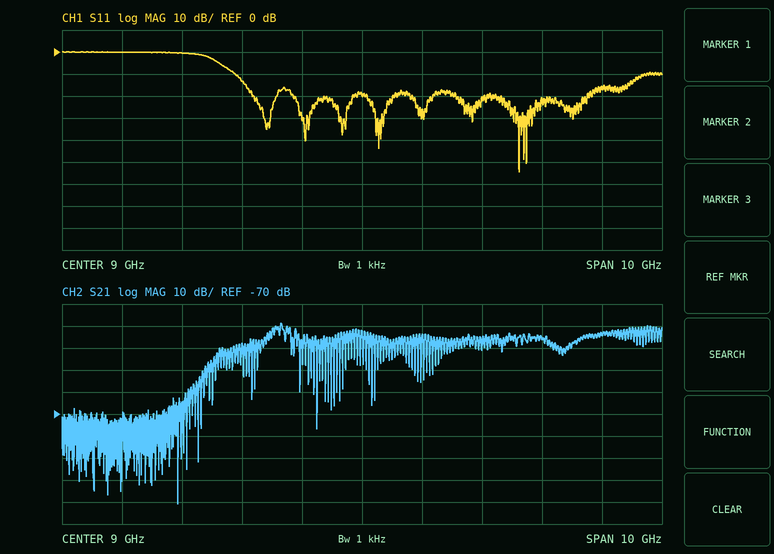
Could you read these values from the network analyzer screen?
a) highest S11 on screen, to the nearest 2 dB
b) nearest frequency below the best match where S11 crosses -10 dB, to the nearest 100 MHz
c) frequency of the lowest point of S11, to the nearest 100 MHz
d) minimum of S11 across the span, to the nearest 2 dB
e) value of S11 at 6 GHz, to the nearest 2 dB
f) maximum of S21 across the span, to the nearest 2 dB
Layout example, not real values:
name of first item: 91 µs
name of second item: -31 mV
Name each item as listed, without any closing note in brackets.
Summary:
highest S11 on screen, to the nearest 2 dB: 0 dB
nearest frequency below the best match where S11 crosses -10 dB, to the nearest 100 MHz: 6.9 GHz
frequency of the lowest point of S11, to the nearest 100 MHz: 11.6 GHz
minimum of S11 across the span, to the nearest 2 dB: -54 dB
value of S11 at 6 GHz, to the nearest 2 dB: 0 dB
maximum of S21 across the span, to the nearest 2 dB: -28 dB
